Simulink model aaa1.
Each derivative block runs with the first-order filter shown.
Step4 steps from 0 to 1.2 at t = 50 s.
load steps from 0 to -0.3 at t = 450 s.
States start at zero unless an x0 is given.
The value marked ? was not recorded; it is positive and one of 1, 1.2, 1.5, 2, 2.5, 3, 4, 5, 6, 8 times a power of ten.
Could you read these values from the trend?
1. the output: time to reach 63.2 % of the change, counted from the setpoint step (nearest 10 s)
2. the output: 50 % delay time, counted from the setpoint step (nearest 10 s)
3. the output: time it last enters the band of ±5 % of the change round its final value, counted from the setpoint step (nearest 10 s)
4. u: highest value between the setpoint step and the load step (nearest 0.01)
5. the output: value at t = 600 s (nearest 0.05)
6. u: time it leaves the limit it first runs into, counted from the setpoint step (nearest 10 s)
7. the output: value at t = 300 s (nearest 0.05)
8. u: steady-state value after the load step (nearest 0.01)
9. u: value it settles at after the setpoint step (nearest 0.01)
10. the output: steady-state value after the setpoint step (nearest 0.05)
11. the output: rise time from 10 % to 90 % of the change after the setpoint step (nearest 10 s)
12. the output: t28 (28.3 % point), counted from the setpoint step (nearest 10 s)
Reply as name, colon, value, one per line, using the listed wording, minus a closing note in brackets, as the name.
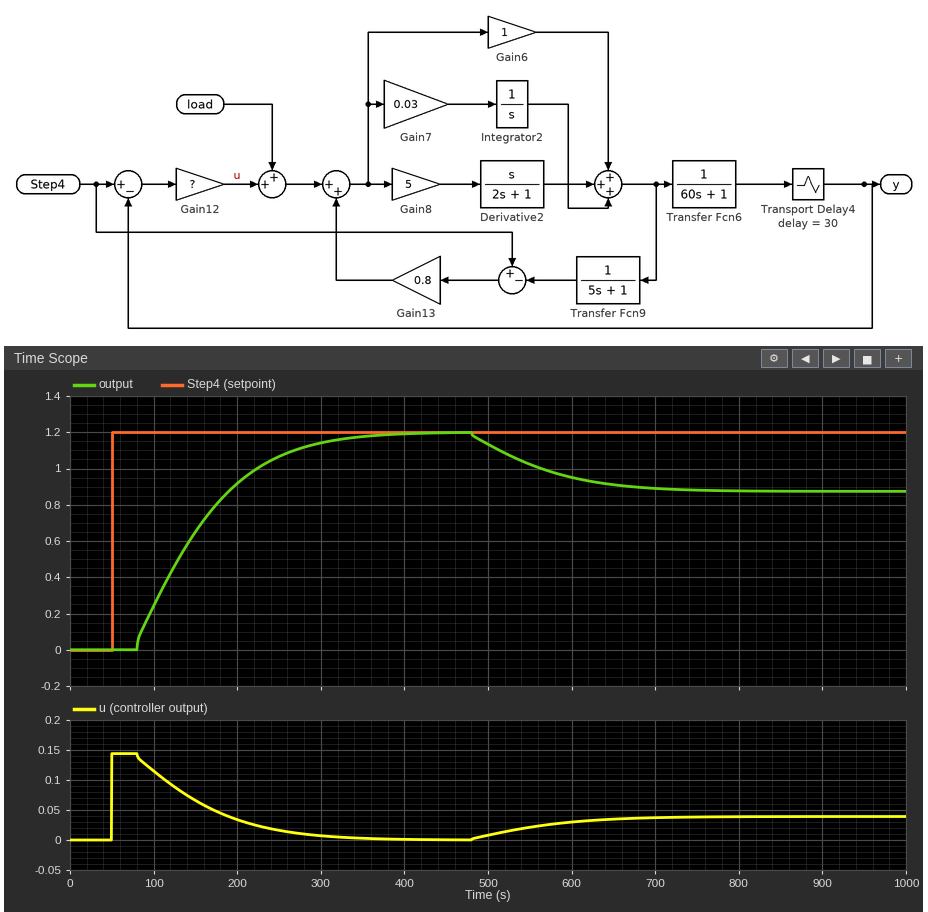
the output: time to reach 63.2 % of the change, counted from the setpoint step: 120 s
the output: 50 % delay time, counted from the setpoint step: 90 s
the output: time it last enters the band of ±5 % of the change round its final value, counted from the setpoint step: 250 s
u: highest value between the setpoint step and the load step: 0.14
the output: value at t = 600 s: 0.95
u: time it leaves the limit it first runs into, counted from the setpoint step: 30 s
the output: value at t = 300 s: 1.15
u: steady-state value after the load step: 0.04
u: value it settles at after the setpoint step: 0.00
the output: steady-state value after the setpoint step: 1.20
the output: rise time from 10 % to 90 % of the change after the setpoint step: 170 s
the output: t28 (28.3 % point), counted from the setpoint step: 60 s
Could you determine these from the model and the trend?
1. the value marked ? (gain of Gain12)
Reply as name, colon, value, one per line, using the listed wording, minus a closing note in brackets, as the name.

the value marked ?: 0.12
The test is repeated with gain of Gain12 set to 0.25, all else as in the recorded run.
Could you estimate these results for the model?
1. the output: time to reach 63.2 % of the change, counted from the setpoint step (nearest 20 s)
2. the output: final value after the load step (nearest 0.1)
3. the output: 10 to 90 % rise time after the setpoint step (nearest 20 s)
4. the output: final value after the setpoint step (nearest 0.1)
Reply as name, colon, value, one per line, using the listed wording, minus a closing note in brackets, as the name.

the output: time to reach 63.2 % of the change, counted from the setpoint step: 100 s
the output: final value after the load step: 0.9
the output: 10 to 90 % rise time after the setpoint step: 140 s
the output: final value after the setpoint step: 1.2
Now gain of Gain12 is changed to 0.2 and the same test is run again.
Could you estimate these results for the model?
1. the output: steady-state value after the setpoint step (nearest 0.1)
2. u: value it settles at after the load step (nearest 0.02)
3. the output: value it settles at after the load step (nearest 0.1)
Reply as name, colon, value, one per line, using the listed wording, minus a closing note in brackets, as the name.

the output: steady-state value after the setpoint step: 1.2
u: value it settles at after the load step: 0.06
the output: value it settles at after the load step: 0.9
